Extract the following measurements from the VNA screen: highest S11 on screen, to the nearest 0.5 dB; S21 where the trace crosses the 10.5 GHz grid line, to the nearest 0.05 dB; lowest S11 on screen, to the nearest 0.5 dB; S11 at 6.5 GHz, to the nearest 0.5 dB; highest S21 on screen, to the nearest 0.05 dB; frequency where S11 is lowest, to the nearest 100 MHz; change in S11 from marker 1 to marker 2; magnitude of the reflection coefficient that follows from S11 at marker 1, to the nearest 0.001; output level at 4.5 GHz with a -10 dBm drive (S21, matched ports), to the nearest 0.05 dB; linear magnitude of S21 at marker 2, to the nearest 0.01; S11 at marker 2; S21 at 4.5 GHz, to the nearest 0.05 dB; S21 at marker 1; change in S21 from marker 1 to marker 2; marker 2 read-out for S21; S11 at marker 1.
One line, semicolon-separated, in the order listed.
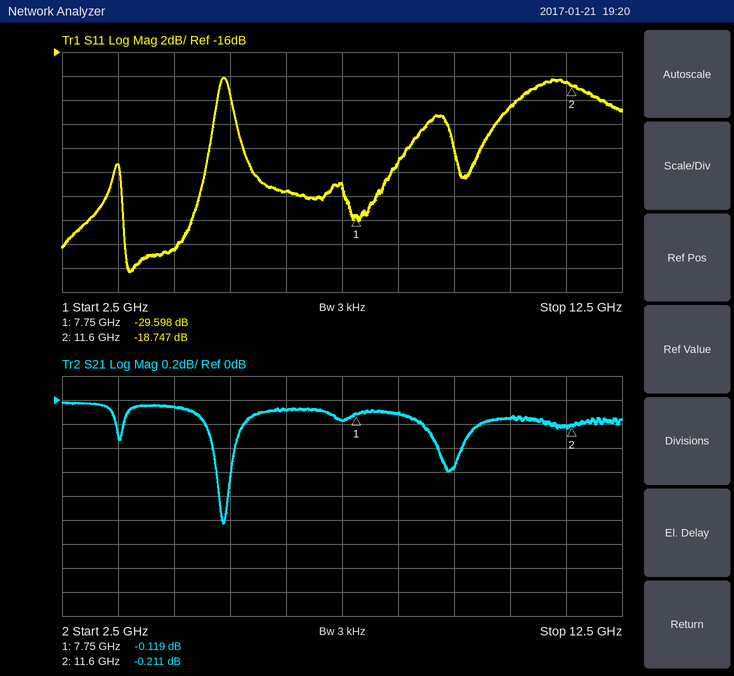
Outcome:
-18.0 dB; -0.15 dB; -34.5 dB; -27.5 dB; 0.00 dB; 3.7 GHz; 10.851 dB; 0.033; -10.05 dBm; 0.98; -18.747 dB; -0.05 dB; -0.119 dB; -0.092 dB; -0.211 dB; -29.598 dB
